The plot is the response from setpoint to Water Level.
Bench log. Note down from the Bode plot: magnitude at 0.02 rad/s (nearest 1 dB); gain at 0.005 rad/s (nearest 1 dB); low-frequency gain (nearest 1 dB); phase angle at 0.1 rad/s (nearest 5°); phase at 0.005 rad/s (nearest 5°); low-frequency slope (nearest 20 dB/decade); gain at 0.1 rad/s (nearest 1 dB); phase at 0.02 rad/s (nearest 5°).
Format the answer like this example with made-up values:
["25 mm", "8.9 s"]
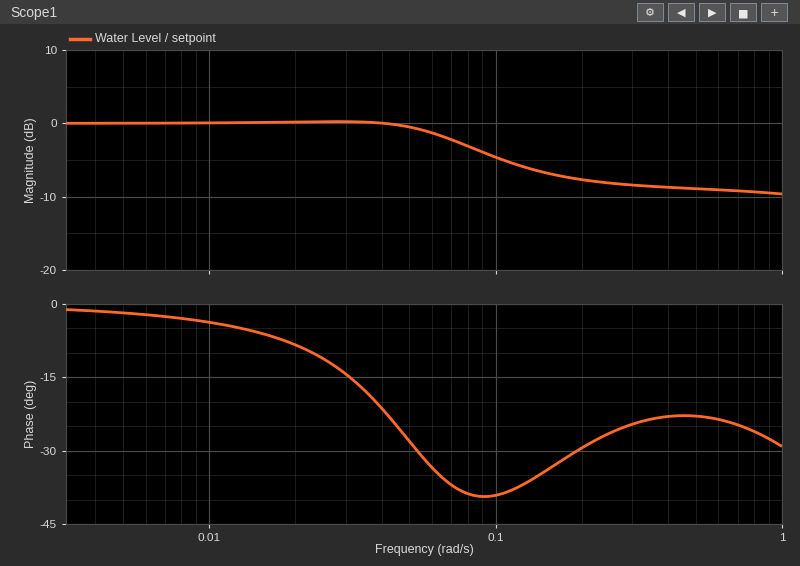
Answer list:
["0 dB", "0 dB", "0 dB", "-40°", "0°", "0 dB/decade", "-5 dB", "-10°"]
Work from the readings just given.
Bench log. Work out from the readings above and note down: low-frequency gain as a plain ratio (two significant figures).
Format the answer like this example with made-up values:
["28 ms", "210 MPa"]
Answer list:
["1.0"]
